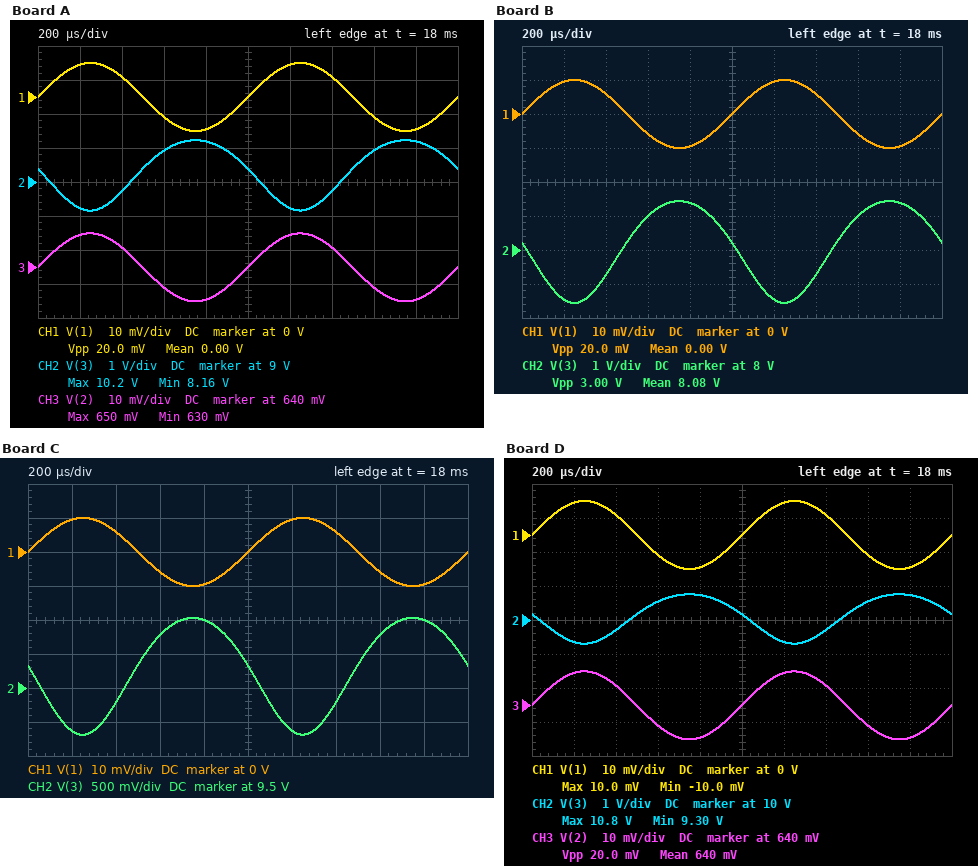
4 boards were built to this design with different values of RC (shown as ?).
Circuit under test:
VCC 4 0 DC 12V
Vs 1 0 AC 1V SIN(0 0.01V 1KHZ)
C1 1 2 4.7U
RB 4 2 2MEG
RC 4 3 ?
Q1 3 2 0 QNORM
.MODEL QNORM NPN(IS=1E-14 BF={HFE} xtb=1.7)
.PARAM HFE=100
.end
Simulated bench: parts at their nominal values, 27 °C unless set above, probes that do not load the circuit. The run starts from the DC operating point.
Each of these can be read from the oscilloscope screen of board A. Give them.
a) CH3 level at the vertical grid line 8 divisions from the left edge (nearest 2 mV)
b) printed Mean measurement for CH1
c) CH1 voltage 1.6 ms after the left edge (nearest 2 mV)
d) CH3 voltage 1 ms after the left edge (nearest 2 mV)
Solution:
634 mV
0.00 V
-6 mV
640 mV
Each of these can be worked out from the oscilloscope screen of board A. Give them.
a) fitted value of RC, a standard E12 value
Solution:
4.7 kΩ
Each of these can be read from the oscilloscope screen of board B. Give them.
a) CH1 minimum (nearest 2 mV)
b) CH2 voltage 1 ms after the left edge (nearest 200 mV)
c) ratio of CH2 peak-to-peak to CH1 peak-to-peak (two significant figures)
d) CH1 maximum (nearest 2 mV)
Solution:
-10 mV
8.2 V
150
10 mV
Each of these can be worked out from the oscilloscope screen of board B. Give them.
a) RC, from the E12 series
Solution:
6.8 kΩ
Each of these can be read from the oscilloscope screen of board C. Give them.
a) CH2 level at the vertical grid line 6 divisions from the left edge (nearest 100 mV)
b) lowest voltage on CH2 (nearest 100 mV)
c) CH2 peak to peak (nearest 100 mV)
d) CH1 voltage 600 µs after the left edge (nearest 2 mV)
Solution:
8.9 V
8.8 V
1.7 V
-6 mV
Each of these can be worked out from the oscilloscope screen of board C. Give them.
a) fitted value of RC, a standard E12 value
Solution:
3.9 kΩ
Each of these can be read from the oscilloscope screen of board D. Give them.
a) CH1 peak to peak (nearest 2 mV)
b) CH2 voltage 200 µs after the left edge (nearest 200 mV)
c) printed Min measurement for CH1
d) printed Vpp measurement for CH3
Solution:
20 mV
9.4 V
-10.0 mV
20.0 mV
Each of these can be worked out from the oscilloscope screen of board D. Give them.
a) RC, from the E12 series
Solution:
3.3 kΩ
